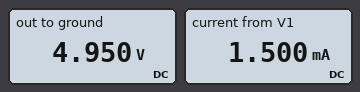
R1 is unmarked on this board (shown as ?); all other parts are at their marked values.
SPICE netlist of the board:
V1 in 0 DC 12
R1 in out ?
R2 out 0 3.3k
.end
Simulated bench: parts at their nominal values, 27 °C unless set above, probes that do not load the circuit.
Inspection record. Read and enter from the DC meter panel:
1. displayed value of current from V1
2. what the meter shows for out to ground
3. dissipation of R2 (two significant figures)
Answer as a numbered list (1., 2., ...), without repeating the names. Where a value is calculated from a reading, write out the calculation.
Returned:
1. 1.500 mA
2. 4.950 V
3. (4.95 V)^2 / 3.3 kΩ = 7.4 mW
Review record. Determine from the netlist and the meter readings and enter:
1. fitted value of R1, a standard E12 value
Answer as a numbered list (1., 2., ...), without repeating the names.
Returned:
1. 4.7 kΩ
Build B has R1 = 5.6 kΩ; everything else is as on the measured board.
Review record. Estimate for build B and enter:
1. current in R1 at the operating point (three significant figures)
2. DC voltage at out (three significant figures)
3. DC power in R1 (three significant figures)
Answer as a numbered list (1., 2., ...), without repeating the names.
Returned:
1. 1.35 mA
2. 4.45 V
3. 10.2 mW
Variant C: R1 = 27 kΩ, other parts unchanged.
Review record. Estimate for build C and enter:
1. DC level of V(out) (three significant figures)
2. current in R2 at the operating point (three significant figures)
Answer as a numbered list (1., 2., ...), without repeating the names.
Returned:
1. 1.31 V
2. 396 µA
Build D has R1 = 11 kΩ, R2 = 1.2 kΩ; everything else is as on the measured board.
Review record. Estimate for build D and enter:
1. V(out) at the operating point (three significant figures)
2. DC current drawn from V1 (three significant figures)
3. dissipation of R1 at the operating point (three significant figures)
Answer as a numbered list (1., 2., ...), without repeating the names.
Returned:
1. 1.18 V
2. 984 µA
3. 10.6 mW
